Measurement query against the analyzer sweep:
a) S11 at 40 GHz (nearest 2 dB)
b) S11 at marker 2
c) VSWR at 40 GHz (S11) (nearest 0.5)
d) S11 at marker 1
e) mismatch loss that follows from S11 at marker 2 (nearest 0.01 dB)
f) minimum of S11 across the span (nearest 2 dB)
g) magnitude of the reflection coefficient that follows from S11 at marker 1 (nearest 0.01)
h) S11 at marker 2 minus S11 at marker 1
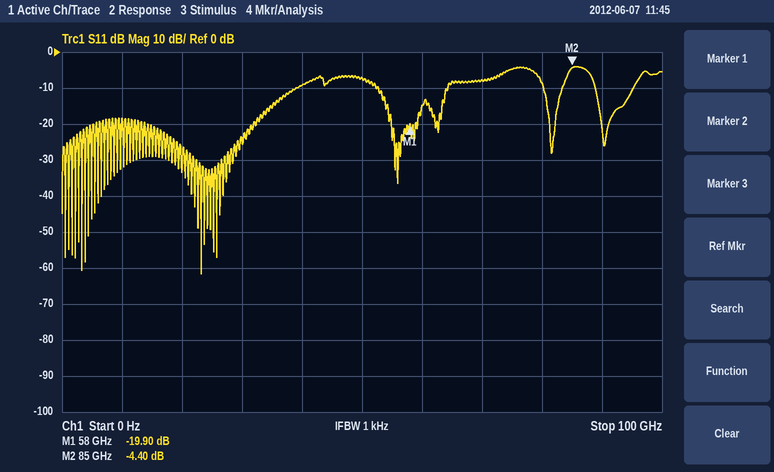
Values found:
-10 dB
-4.40 dB
2.0
-19.90 dB
1.96 dB
-62 dB
0.10
15.50 dB
